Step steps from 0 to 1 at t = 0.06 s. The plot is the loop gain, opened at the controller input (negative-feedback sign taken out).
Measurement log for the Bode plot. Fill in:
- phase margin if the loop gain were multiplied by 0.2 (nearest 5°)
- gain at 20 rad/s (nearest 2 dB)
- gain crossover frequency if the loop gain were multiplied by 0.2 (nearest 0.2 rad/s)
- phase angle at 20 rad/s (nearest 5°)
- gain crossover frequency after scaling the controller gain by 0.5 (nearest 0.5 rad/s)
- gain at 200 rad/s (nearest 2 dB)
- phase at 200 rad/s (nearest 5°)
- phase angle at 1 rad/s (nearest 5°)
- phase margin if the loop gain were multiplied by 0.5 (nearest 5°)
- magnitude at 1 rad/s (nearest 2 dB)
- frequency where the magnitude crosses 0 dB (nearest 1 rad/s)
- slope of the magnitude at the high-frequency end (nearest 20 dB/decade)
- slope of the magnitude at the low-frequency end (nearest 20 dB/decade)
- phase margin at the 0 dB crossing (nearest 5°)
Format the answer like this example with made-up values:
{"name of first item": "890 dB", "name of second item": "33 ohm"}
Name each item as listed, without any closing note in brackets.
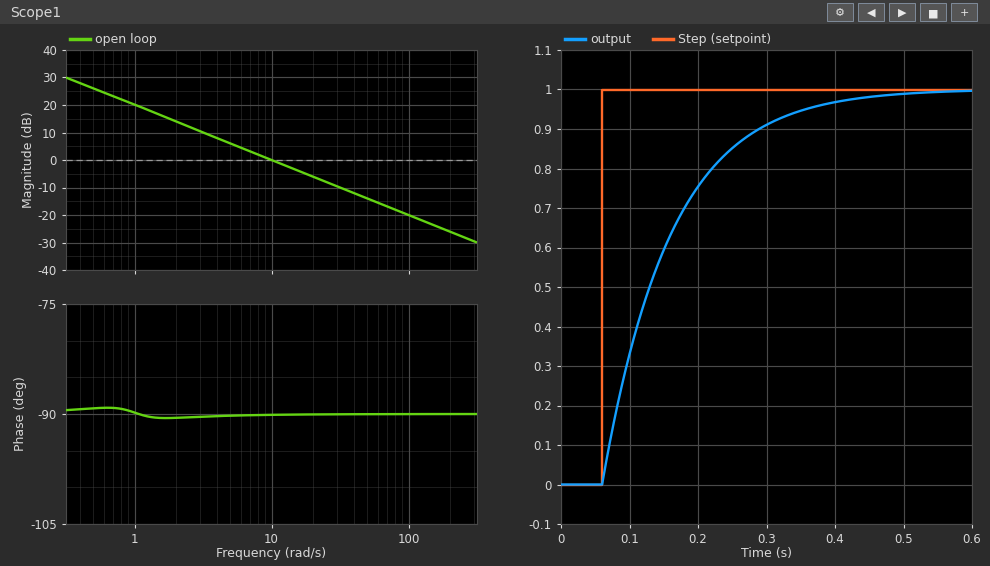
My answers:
{"phase margin if the loop gain were multiplied by 0.2": "90°", "gain at 20 rad/s": "-6 dB", "gain crossover frequency if the loop gain were multiplied by 0.2": "2.0 rad/s", "phase angle at 20 rad/s": "-90°", "gain crossover frequency after scaling the controller gain by 0.5": "5.0 rad/s", "gain at 200 rad/s": "-26 dB", "phase at 200 rad/s": "-90°", "phase angle at 1 rad/s": "-90°", "phase margin if the loop gain were multiplied by 0.5": "90°", "magnitude at 1 rad/s": "20 dB", "frequency where the magnitude crosses 0 dB": "10 rad/s", "slope of the magnitude at the high-frequency end": "-20 dB/decade", "slope of the magnitude at the low-frequency end": "-20 dB/decade", "phase margin at the 0 dB crossing": "90°"}
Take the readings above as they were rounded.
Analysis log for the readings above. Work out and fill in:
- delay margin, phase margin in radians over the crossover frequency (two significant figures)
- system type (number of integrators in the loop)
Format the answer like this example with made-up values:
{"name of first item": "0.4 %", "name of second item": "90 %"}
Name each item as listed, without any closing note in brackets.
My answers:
{"delay margin, phase margin in radians over the crossover frequency": "0.16 s", "system type": "1"}
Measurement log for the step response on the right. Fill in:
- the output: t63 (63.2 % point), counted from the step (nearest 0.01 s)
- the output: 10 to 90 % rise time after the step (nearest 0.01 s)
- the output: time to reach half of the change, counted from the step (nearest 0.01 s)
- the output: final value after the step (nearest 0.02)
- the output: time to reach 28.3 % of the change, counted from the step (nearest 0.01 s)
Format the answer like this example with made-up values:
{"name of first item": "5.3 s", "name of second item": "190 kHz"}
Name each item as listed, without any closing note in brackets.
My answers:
{"the output: t63 (63.2 % point), counted from the step": "0.10 s", "the output: 10 to 90 % rise time after the step": "0.22 s", "the output: time to reach half of the change, counted from the step": "0.07 s", "the output: final value after the step": "1.00", "the output: time to reach 28.3 % of the change, counted from the step": "0.03 s"}
